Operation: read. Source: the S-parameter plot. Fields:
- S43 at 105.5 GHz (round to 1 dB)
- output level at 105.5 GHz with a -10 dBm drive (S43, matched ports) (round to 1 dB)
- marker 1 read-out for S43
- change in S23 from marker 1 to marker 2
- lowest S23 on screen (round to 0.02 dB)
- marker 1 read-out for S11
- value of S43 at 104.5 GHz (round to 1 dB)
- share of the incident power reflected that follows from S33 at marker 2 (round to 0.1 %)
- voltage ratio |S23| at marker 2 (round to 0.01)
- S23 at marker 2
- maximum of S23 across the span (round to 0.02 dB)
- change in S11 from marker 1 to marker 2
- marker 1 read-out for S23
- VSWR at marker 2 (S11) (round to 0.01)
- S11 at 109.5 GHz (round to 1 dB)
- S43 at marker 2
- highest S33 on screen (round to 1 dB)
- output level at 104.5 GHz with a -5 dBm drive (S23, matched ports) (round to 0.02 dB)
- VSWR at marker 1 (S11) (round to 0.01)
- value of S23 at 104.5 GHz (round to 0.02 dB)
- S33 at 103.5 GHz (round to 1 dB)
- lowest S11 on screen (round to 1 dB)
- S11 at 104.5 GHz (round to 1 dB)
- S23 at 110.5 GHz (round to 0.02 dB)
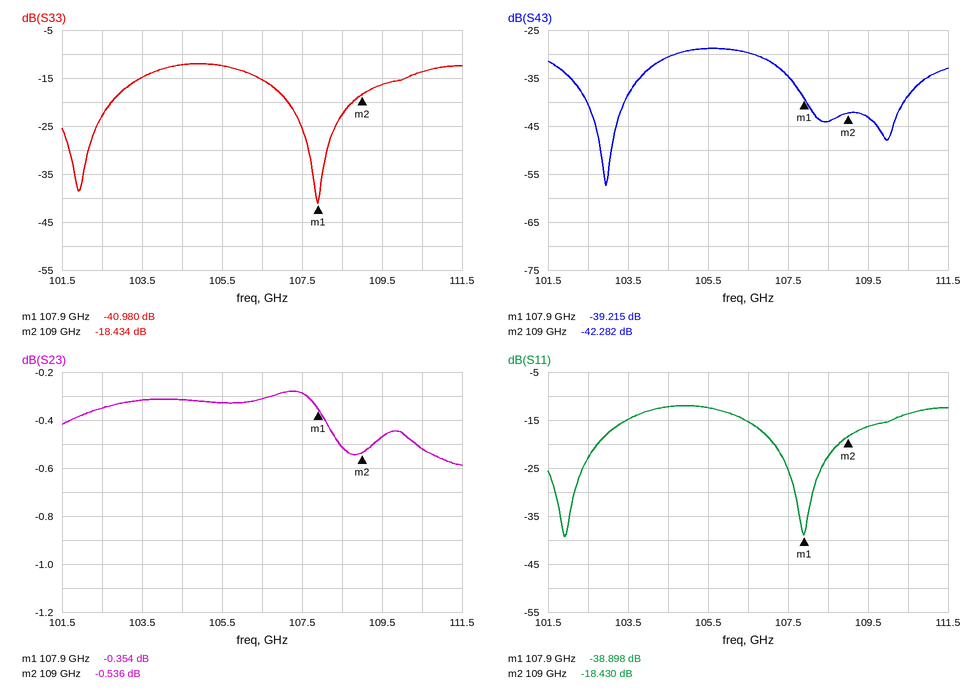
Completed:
-29 dB
-39 dBm
-39.215 dB
-0.182 dB
-0.58 dB
-38.898 dB
-31 dB
1.4 %
0.94
-0.536 dB
-0.28 dB
20.468 dB
-0.354 dB
1.27
-16 dB
-42.282 dB
-12 dB
-5.32 dBm
1.02
-0.32 dB
-15 dB
-39 dB
-12 dB
-0.52 dB
